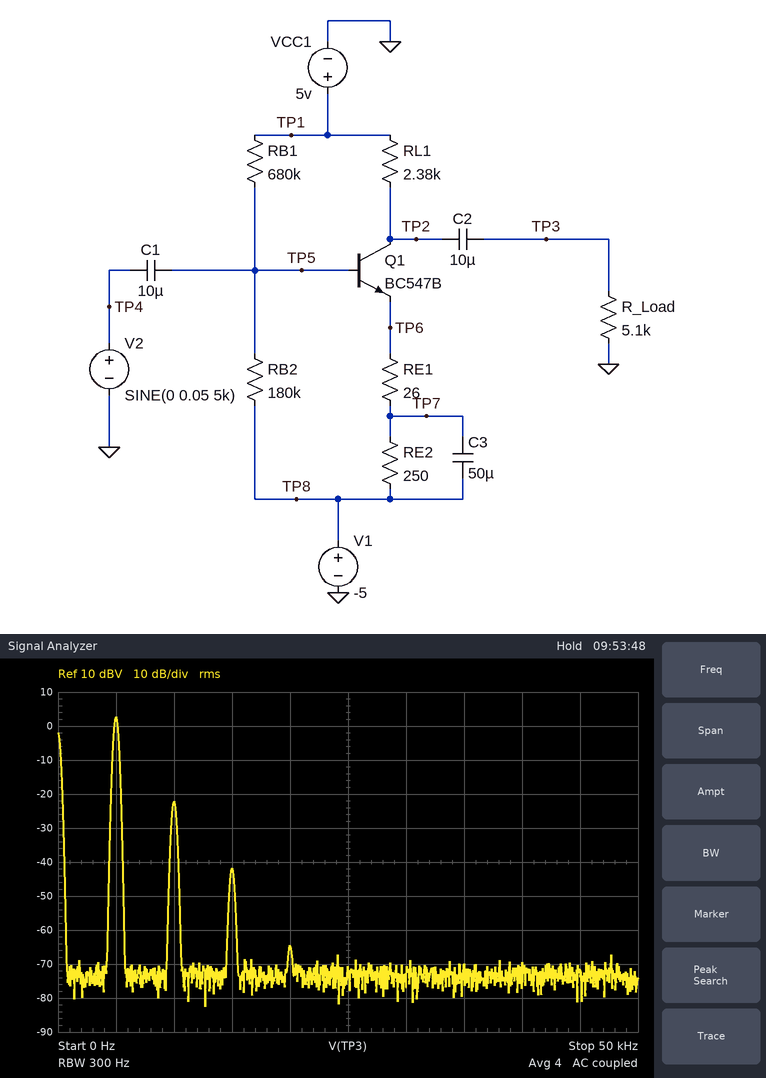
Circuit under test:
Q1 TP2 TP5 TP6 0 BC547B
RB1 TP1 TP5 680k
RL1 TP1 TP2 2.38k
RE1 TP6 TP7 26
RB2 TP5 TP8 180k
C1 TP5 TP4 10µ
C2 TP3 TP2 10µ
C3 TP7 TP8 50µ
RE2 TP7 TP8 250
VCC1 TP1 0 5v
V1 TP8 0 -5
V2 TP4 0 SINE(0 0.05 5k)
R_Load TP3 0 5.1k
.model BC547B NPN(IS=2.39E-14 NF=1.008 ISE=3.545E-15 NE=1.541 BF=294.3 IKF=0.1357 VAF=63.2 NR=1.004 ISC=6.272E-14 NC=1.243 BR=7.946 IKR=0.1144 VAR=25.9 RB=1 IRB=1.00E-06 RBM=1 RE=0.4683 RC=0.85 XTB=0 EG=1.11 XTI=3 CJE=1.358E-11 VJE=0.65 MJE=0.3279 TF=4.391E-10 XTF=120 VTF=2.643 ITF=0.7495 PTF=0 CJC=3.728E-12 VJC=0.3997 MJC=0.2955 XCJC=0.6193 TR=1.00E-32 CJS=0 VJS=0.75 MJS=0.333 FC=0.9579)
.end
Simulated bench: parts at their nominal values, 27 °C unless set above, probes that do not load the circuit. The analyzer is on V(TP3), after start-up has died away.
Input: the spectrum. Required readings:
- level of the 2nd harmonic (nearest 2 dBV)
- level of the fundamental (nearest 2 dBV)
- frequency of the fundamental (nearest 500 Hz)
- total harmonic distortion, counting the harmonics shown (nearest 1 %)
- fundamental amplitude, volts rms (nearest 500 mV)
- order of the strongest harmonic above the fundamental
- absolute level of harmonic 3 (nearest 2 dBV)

-22 dBV
2 dBV
5.0 kHz
6 %
1.5 V
2
-42 dBV
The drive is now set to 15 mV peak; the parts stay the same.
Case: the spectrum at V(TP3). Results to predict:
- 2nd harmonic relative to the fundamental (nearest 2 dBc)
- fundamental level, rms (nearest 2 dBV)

-36 dBc
-8 dBV
